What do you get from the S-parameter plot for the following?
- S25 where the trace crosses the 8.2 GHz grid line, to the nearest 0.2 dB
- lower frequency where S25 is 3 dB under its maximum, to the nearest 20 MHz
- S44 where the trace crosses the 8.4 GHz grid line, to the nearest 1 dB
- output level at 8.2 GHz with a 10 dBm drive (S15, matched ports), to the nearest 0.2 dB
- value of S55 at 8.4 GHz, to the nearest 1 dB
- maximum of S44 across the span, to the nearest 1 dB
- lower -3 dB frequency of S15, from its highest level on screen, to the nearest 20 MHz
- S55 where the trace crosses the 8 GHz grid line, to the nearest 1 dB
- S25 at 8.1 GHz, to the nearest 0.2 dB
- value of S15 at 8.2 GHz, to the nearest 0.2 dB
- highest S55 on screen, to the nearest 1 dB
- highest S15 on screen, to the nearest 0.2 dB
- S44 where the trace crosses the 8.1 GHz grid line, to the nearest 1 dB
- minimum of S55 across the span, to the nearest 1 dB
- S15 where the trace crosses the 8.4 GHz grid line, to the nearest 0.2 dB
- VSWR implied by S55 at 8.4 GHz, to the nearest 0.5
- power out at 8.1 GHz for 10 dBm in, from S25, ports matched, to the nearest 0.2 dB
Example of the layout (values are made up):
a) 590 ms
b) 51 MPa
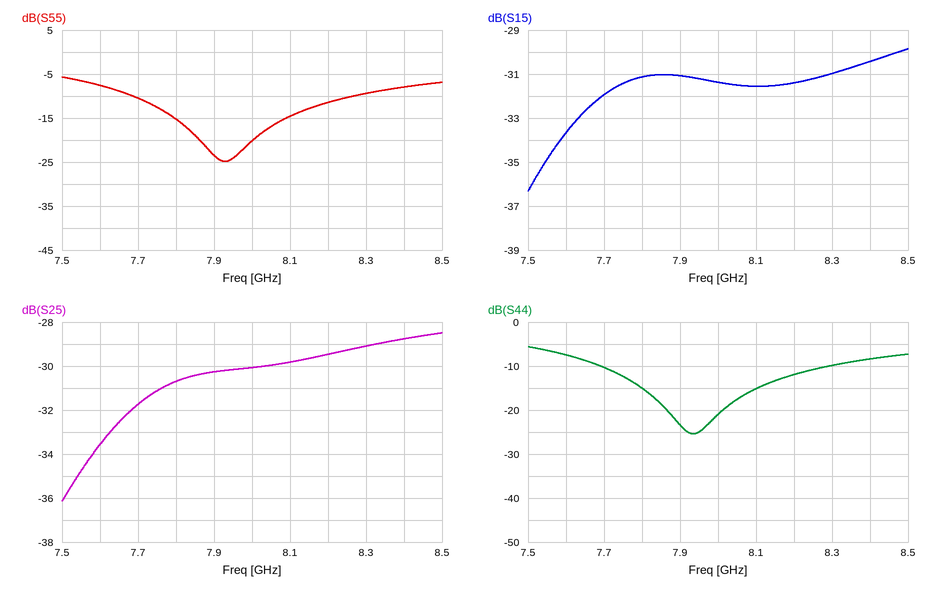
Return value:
a) -29.4 dB
b) 7.72 GHz
c) -8 dB
d) -21.4 dBm
e) -8 dB
f) -6 dB
g) 7.64 GHz
h) -20 dB
i) -29.8 dB
j) -31.4 dB
k) -6 dB
l) -29.8 dB
m) -15 dB
n) -25 dB
o) -30.4 dB
p) 2.5
q) -19.8 dBm
